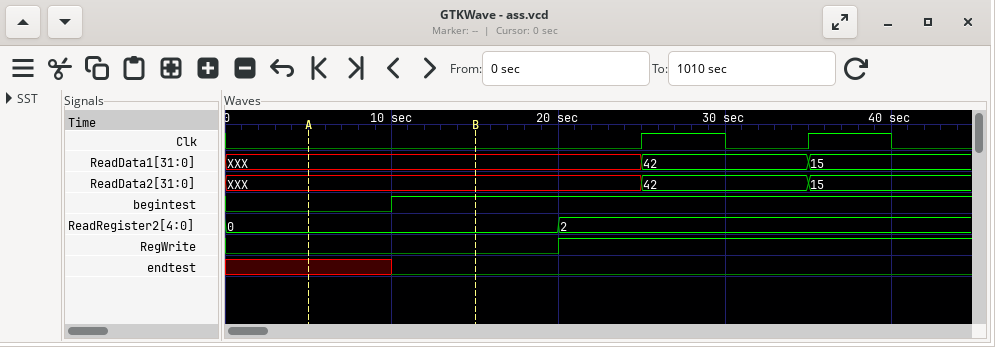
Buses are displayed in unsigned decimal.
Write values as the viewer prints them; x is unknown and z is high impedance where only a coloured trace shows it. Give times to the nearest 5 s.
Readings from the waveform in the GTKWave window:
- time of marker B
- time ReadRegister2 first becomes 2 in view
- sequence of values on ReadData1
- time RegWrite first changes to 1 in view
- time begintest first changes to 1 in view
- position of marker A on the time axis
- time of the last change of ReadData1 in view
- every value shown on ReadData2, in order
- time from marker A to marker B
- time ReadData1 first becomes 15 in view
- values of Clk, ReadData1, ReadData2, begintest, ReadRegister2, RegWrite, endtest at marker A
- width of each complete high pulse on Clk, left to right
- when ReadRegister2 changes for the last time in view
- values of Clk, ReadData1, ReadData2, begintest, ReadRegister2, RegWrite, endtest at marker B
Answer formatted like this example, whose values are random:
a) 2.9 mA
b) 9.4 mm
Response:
a) 15 s
b) 20 s
c) XXX, 42, 15
d) 20 s
e) 10 s
f) 5 s
g) 35 s
h) XXX, 42, 15
i) 10 s
j) 35 s
k) Clk=0, ReadData1=XXX, ReadData2=XXX, begintest=0, ReadRegister2=0, RegWrite=0, endtest=x
l) 5 s, 5 s
m) 20 s
n) Clk=0, ReadData1=XXX, ReadData2=XXX, begintest=1, ReadRegister2=0, RegWrite=0, endtest=0
